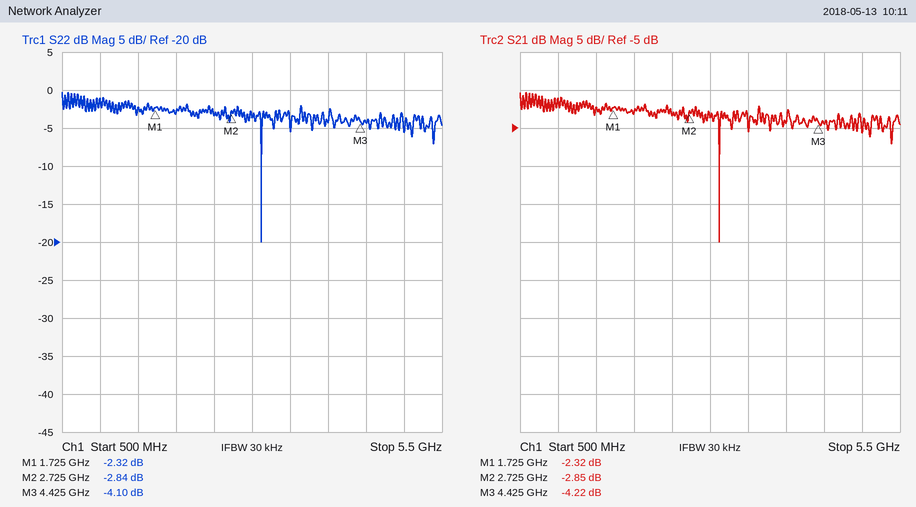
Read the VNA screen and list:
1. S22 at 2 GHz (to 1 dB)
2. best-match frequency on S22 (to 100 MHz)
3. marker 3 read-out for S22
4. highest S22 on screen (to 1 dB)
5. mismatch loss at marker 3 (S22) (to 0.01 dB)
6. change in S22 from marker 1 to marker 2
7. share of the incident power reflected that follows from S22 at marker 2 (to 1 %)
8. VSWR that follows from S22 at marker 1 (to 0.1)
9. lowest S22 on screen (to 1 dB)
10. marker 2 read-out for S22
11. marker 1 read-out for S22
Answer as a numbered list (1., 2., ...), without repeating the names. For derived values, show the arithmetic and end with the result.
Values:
1. -3 dB
2. 3.1 GHz
3. -4.10 dB
4. 0 dB
5. −10 log10(1 − 10^(-4.1/10)) ≈ 2.14 dB
6. -2.84 − (-2.32) = -0.52 dB
7. 10^(-2.84/10) ≈ 52 %
8. (1 + 0.7656)/(1 − 0.7656) ≈ 7.5
9. -20 dB
10. -2.84 dB
11. -2.32 dB
